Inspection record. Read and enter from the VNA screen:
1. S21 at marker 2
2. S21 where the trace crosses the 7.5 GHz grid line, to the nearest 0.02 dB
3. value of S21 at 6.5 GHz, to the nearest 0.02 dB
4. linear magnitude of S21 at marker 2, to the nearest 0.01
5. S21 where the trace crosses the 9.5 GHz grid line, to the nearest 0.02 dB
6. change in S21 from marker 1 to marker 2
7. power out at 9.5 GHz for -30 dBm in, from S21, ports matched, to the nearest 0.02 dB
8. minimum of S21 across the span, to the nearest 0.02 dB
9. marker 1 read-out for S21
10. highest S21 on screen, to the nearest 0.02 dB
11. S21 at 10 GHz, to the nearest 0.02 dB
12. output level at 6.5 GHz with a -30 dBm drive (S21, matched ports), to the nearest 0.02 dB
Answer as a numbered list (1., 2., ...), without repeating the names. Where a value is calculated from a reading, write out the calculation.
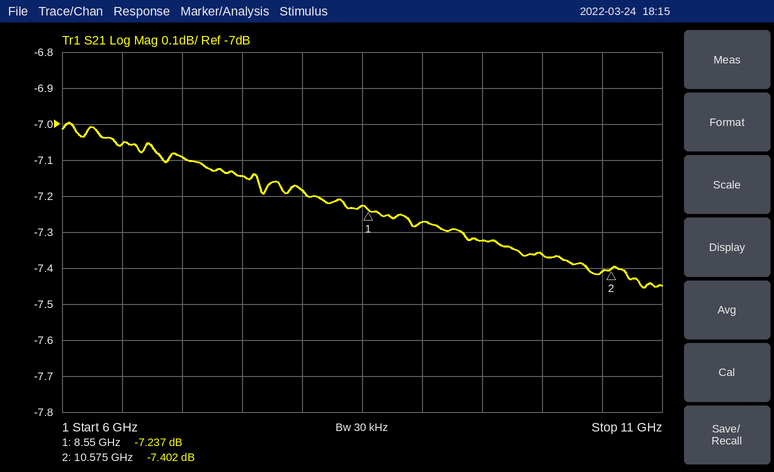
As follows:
1. -7.402 dB
2. -7.14 dB
3. -7.06 dB
4. 10^(-7.402/20) ≈ 0.43
5. -7.32 dB
6. -7.402 − (-7.237) = -0.165 dB
7. -30 dBm + (-7.32 dB) = -37.32 dBm
8. -7.46 dB
9. -7.237 dB
10. -7.00 dB
11. -7.36 dB
12. -30 dBm + (-7.06 dB) = -37.06 dBm
